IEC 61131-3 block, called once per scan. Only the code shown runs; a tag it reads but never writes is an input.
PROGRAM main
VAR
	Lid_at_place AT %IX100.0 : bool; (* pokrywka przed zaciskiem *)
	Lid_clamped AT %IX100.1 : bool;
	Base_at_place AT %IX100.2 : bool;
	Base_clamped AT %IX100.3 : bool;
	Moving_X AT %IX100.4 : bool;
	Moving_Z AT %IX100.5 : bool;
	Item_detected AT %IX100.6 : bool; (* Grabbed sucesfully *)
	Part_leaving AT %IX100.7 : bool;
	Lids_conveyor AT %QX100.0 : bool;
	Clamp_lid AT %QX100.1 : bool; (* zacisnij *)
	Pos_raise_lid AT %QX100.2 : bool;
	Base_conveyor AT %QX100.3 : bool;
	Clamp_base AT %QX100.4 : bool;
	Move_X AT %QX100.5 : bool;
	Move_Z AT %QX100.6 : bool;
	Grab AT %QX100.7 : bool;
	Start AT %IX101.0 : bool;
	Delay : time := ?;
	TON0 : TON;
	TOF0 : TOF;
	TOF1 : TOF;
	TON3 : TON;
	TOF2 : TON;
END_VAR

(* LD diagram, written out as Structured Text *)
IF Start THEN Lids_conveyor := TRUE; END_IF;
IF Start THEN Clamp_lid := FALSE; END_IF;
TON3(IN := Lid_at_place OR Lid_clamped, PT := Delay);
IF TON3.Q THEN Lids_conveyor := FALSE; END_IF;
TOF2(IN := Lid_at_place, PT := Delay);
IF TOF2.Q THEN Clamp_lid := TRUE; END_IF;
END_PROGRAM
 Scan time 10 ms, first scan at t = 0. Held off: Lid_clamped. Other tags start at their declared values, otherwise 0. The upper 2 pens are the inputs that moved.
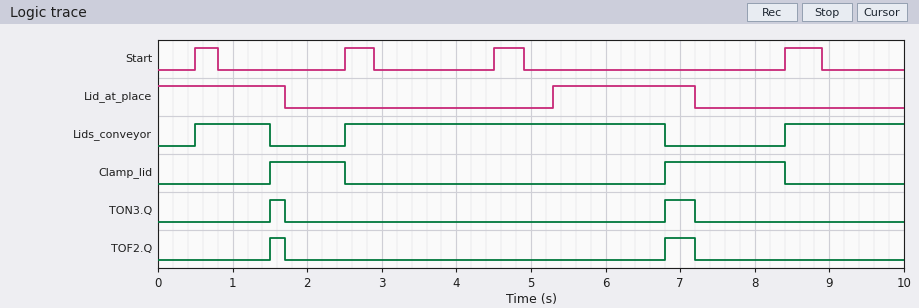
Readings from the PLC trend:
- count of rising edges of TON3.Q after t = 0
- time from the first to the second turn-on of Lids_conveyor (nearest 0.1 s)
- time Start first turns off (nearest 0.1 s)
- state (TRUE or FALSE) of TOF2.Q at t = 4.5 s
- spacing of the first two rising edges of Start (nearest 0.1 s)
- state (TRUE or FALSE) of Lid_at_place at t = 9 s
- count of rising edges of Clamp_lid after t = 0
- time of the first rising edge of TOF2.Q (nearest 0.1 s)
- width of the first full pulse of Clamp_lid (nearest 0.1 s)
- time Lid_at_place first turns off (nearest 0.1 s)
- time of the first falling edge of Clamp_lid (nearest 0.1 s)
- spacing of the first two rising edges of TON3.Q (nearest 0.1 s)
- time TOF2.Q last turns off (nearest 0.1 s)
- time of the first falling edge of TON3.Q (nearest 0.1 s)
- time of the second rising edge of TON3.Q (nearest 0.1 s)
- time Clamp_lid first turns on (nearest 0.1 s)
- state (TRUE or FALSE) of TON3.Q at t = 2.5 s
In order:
2
2.0 s
0.8 s
FALSE
2.0 s
FALSE
2
1.5 s
1.0 s
1.7 s
2.5 s
5.3 s
7.2 s
1.7 s
6.8 s
1.5 s
FALSE
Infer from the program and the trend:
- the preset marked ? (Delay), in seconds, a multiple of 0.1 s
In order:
1.5 s
